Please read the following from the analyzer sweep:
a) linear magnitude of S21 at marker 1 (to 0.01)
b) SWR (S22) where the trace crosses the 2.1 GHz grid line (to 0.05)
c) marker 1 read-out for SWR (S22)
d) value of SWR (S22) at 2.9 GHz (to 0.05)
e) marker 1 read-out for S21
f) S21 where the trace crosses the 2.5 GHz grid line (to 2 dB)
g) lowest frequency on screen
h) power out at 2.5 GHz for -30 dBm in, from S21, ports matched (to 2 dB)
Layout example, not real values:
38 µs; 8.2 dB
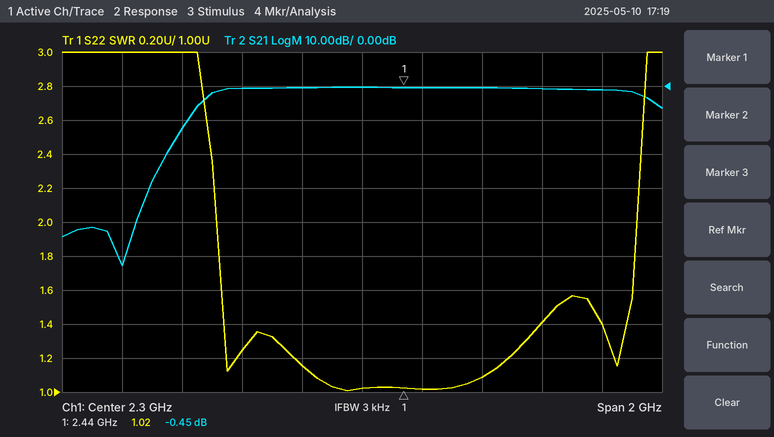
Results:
0.95; 1.15; 1.02; 1.40; -0.45 dB; 0 dB; 1.3 GHz; -30 dBm
